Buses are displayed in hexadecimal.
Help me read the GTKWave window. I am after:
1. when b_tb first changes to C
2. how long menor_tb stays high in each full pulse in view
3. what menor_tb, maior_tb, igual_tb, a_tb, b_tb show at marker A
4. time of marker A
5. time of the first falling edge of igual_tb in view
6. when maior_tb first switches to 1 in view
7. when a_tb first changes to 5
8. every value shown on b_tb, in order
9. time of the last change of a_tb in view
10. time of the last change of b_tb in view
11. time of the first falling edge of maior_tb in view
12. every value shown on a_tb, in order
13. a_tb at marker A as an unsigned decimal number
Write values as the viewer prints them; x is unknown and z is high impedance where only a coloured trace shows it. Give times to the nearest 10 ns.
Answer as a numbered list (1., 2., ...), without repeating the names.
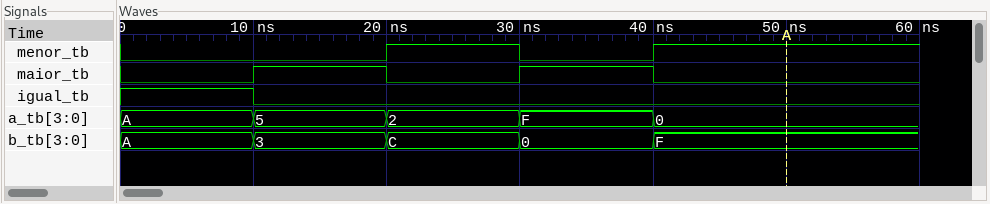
1. 20 ns
2. 10 ns
3. menor_tb=1, maior_tb=0, igual_tb=0, a_tb=0, b_tb=F
4. 50 ns
5. 10 ns
6. 10 ns
7. 10 ns
8. A, 3, C, 0, F
9. 40 ns
10. 40 ns
11. 20 ns
12. A, 5, 2, F, 0
13. 0
